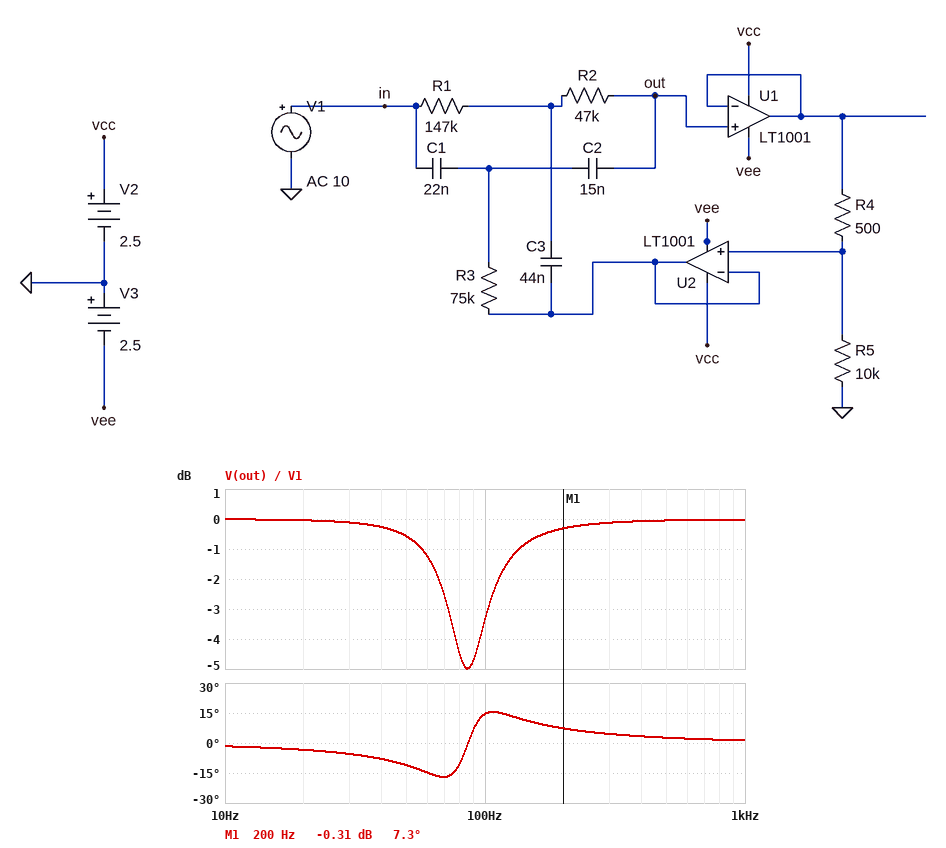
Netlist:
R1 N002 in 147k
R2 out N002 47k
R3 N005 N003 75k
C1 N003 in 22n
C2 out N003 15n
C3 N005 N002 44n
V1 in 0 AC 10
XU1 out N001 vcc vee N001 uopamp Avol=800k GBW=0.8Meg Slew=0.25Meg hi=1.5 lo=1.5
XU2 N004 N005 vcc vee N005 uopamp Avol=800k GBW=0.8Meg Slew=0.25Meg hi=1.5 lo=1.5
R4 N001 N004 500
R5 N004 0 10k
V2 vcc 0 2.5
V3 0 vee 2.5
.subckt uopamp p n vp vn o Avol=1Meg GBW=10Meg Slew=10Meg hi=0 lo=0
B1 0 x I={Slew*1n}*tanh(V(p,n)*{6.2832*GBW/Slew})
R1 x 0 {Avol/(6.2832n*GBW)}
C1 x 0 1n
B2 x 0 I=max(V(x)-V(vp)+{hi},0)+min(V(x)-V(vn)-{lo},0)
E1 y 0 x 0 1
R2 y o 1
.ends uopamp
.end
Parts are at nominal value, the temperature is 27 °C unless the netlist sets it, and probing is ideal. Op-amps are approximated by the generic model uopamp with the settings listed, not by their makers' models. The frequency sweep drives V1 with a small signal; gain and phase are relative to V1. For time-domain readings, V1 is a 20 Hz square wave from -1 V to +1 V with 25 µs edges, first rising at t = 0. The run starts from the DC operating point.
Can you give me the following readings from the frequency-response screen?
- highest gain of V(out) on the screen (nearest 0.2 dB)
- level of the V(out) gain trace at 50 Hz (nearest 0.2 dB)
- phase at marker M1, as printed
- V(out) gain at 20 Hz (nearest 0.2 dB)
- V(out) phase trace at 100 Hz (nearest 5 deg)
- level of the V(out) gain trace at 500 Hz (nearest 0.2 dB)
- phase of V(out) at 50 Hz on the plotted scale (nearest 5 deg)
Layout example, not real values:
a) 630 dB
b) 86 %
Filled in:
a) 0 dB
b) -0.6 dB
c) 7.3 deg
d) 0 dB
e) 15 deg
f) 0 dB
g) -10 deg
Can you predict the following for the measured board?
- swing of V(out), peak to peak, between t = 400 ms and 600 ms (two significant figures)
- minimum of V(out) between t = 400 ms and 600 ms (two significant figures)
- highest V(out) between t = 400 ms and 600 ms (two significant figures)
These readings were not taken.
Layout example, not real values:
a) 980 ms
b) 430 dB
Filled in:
a) 2.1 V
b) -1.0 V
c) 1.0 V
